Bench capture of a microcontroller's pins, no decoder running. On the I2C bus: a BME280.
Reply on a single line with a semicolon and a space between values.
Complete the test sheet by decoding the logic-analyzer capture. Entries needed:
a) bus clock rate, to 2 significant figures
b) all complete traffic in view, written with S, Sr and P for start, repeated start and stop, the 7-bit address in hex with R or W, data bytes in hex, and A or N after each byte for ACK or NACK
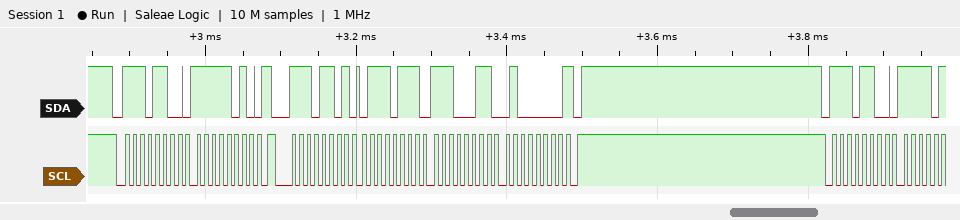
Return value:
100 kHz; S 76W A FA A Sr 76R A 77 A E3 A 40 N P S 76W A
